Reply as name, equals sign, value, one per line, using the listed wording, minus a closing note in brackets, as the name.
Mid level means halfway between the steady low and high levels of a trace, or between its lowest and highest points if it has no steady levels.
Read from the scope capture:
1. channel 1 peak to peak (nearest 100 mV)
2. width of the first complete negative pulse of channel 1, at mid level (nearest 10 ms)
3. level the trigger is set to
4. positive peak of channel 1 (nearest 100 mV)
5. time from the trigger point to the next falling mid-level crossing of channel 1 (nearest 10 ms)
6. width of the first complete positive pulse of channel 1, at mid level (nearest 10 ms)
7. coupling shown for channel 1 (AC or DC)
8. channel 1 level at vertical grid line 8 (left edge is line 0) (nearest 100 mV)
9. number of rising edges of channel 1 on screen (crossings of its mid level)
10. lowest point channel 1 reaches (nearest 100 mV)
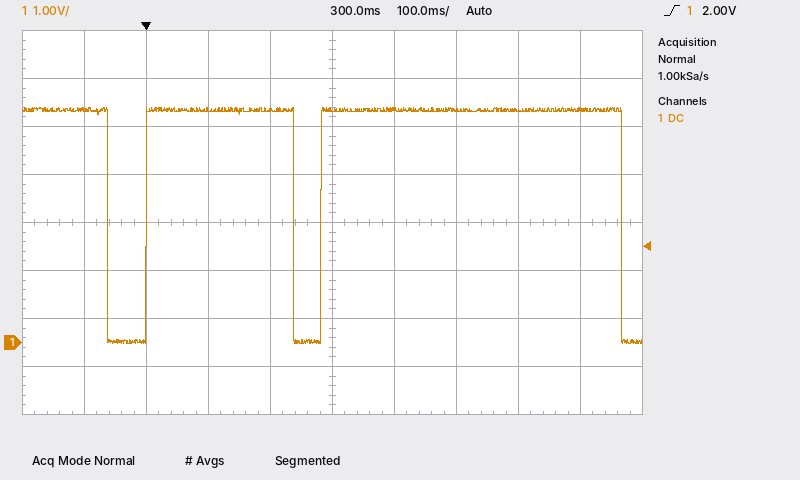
channel 1 peak to peak = 4.9 V
width of the first complete negative pulse of channel 1, at mid level = 60 ms
level the trigger is set to = 2.00 V
positive peak of channel 1 = 4.9 V
time from the trigger point to the next falling mid-level crossing of channel 1 = 240 ms
width of the first complete positive pulse of channel 1, at mid level = 240 ms
coupling shown for channel 1 = DC
channel 1 level at vertical grid line 8 (left edge is line 0) = 4.8 V
number of rising edges of channel 1 on screen = 2
lowest point channel 1 reaches = 0.0 V
